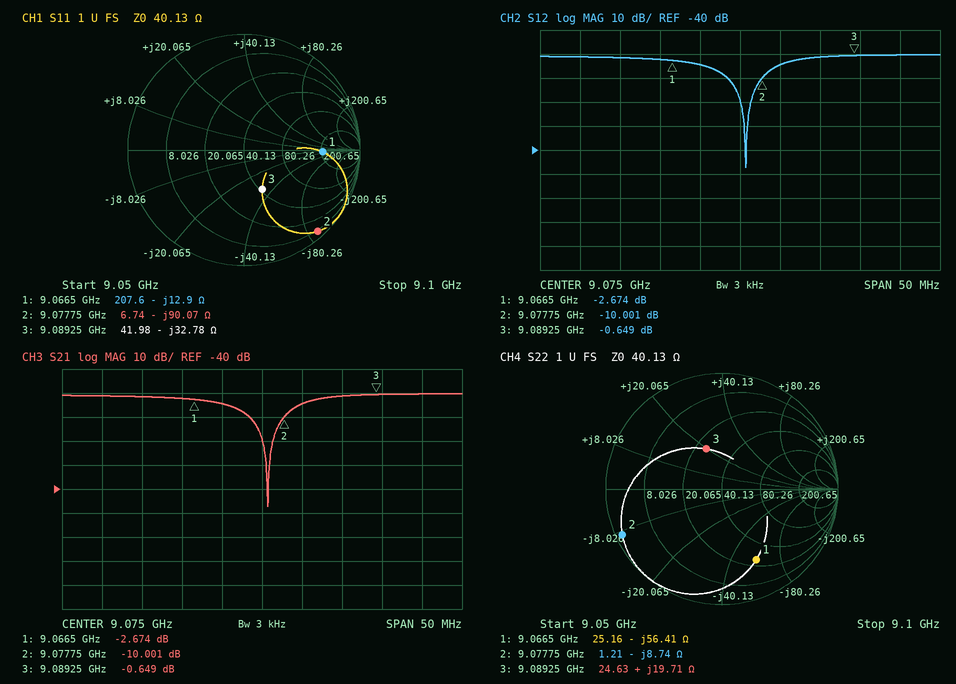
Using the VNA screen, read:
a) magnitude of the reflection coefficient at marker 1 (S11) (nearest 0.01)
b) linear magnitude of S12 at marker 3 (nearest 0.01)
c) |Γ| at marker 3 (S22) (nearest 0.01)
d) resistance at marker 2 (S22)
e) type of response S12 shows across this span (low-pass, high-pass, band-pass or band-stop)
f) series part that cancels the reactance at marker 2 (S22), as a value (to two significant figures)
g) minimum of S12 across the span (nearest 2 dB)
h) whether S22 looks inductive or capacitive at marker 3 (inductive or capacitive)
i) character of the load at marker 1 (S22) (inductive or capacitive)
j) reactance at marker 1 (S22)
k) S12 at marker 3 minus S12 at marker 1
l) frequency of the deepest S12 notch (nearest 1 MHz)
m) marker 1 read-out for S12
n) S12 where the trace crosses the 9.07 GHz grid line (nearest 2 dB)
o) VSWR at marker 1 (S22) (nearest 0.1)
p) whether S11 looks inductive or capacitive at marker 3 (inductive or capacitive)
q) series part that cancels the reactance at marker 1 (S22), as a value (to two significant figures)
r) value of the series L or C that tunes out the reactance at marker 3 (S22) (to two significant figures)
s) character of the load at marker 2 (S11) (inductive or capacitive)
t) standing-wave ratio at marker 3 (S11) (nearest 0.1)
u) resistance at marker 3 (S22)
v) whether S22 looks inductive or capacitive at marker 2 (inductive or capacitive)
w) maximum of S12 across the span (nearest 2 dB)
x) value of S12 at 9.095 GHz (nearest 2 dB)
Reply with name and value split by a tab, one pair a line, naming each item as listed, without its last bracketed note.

magnitude of the reflection coefficient at marker 1 (S11)	0.68
linear magnitude of S12 at marker 3	0.93
|Γ| at marker 3 (S22)	0.37
resistance at marker 2	1.21 Ω
type of response S12 shows across this span	band-stop
series part that cancels the reactance at marker 2 (S22), as a value	150 pH
minimum of S12 across the span	-48 dB
whether S22 looks inductive or capacitive at marker 3	inductive
character of the load at marker 1 (S22)	capacitive
reactance at marker 1	-56.41 Ω
S12 at marker 3 minus S12 at marker 1	2.025 dB
frequency of the deepest S12 notch	9.076 GHz
marker 1 read-out for S12	-2.674 dB
S12 where the trace crosses the 9.07 GHz grid line	-4 dB
VSWR at marker 1 (S22)	5.2
whether S11 looks inductive or capacitive at marker 3	capacitive
series part that cancels the reactance at marker 1 (S22), as a value	990 pH
value of the series L or C that tunes out the reactance at marker 3 (S22)	890 fF
character of the load at marker 2 (S11)	capacitive
standing-wave ratio at marker 3 (S11)	2.2
resistance at marker 3	24.63 Ω
whether S22 looks inductive or capacitive at marker 2	capacitive
maximum of S12 across the span	0 dB
value of S12 at 9.095 GHz	0 dB
